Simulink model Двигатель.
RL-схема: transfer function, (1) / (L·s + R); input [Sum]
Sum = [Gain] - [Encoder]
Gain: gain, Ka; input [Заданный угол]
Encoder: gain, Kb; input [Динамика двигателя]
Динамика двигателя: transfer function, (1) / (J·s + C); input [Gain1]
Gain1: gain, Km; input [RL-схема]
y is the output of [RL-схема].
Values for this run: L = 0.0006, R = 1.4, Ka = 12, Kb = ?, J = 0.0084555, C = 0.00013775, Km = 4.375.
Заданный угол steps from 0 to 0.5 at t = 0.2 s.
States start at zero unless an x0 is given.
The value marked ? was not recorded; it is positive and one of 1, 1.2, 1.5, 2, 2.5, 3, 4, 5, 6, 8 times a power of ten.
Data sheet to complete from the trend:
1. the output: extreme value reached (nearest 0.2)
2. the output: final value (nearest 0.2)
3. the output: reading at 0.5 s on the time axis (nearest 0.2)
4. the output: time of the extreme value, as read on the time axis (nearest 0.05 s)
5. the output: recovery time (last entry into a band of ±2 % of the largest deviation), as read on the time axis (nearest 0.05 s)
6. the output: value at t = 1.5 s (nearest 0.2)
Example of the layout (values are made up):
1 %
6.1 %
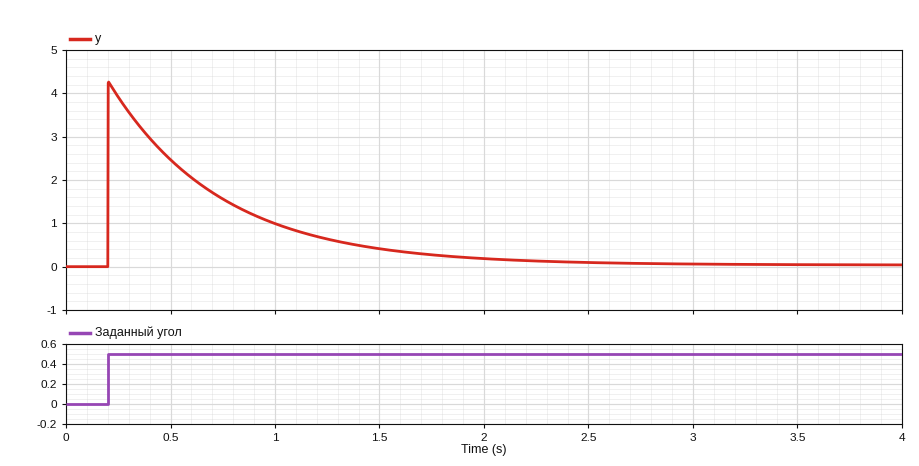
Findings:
4.2
0.0
2.4
0.20 s
2.30 s
0.4
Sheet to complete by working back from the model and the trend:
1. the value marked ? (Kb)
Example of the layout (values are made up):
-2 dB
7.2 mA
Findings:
0.005
